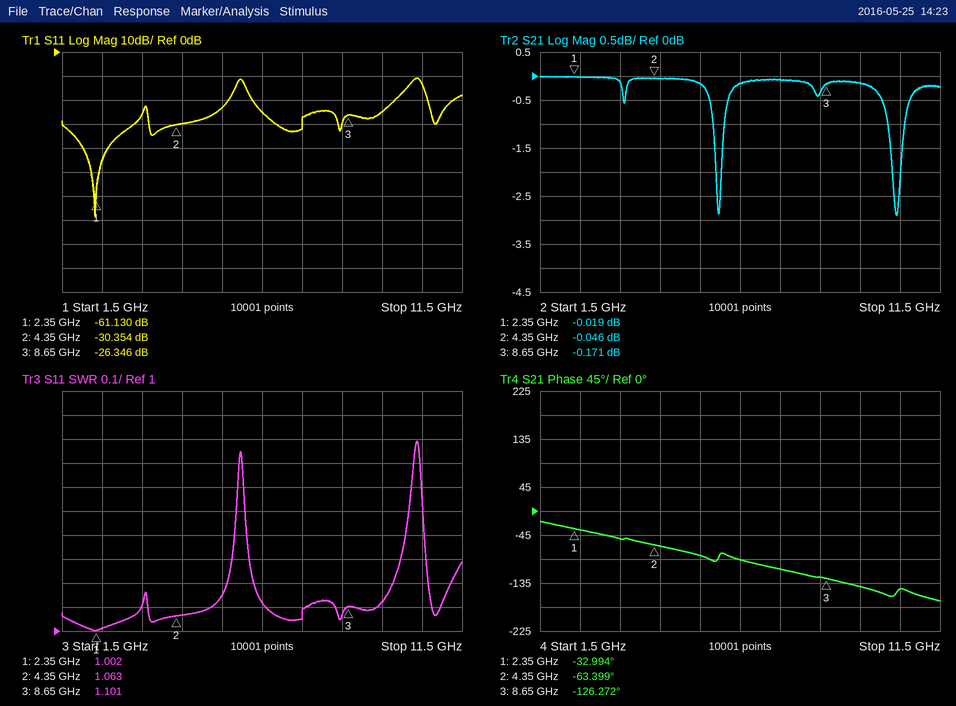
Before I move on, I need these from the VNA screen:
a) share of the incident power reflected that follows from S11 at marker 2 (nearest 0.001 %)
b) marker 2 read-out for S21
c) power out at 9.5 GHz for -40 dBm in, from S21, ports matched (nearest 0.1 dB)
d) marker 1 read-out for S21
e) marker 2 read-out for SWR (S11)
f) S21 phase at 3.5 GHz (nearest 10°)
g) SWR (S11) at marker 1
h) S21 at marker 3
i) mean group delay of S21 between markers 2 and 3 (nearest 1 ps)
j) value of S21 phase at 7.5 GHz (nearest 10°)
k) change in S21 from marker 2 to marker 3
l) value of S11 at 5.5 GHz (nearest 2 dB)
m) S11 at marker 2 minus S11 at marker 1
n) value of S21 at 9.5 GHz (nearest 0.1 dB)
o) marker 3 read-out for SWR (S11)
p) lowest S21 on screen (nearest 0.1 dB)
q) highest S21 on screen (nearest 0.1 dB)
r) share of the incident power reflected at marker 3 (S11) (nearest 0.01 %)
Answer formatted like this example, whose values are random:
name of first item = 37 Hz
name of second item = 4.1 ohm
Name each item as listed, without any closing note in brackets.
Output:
share of the incident power reflected that follows from S11 at marker 2 = 0.092 %
marker 2 read-out for S21 = -0.046 dB
power out at 9.5 GHz for -40 dBm in, from S21, ports matched = -40.1 dBm
marker 1 read-out for S21 = -0.019 dB
marker 2 read-out for SWR = 1.063
S21 phase at 3.5 GHz = -50°
SWR (S11) at marker 1 = 1.002
S21 at marker 3 = -0.171 dB
mean group delay of S21 between markers 2 and 3 = 41 ps
value of S21 phase at 7.5 GHz = -110°
change in S21 from marker 2 to marker 3 = -0.125 dB
value of S11 at 5.5 GHz = -24 dB
S11 at marker 2 minus S11 at marker 1 = 30.776 dB
value of S21 at 9.5 GHz = -0.1 dB
marker 3 read-out for SWR = 1.101
lowest S21 on screen = -2.9 dB
highest S21 on screen = 0.0 dB
share of the incident power reflected at marker 3 (S11) = 0.23 %
